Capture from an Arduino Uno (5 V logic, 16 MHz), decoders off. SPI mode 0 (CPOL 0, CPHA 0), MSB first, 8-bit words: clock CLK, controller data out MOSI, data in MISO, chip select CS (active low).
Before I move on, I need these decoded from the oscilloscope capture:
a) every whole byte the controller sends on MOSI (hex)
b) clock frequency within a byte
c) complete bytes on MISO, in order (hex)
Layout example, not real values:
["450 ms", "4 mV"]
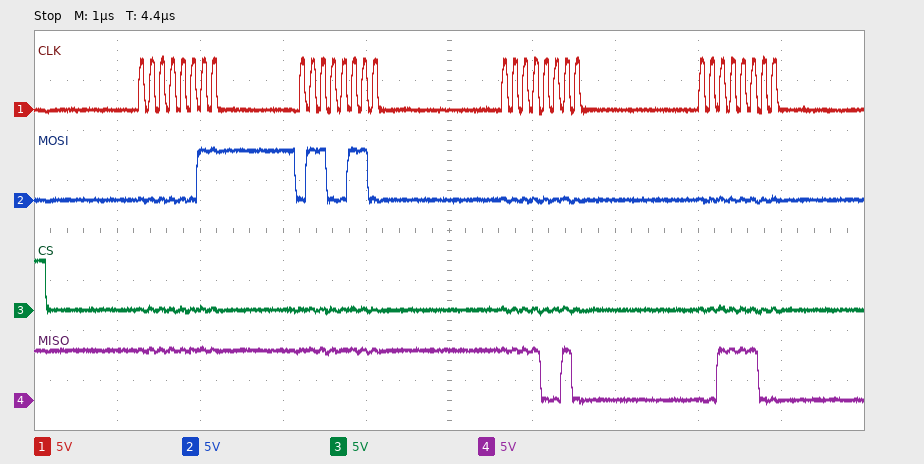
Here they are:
["03 66 00 00", "8 MHz", "FF FF F2 3C"]
